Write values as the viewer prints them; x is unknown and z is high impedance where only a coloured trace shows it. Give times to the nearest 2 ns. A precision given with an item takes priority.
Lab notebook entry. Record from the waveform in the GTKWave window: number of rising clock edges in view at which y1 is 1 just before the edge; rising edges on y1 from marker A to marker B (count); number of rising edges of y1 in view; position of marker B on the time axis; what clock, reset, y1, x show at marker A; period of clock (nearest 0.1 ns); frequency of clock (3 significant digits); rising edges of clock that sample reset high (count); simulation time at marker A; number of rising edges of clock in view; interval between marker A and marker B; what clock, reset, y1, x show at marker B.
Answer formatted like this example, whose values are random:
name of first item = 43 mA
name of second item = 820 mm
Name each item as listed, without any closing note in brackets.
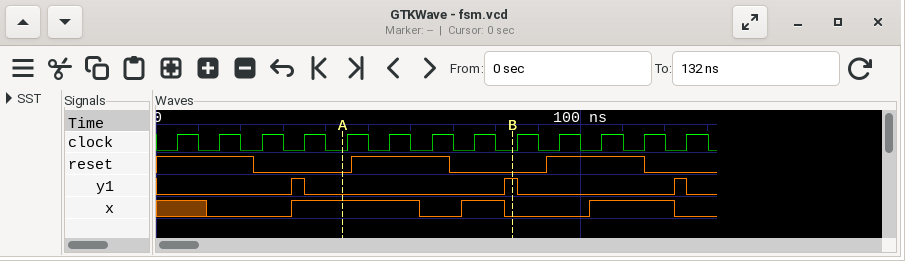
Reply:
number of rising clock edges in view at which y1 is 1 just before the edge = 3
rising edges on y1 from marker A to marker B = 1
number of rising edges of y1 in view = 3
position of marker B on the time axis = 84 ns
what clock, reset, y1, x show at marker A = clock=0, reset=0, y1=0, x=1
period of clock = 10 ns
frequency of clock = 100 MHz
rising edges of clock that sample reset high = 7
simulation time at marker A = 44 ns
number of rising edges of clock in view = 13
interval between marker A and marker B = 40 ns
what clock, reset, y1, x show at marker B = clock=0, reset=0, y1=1, x=0
